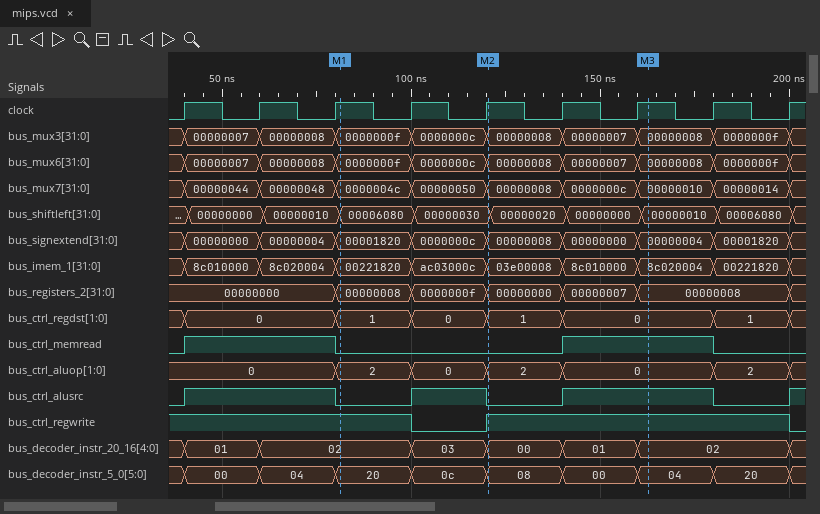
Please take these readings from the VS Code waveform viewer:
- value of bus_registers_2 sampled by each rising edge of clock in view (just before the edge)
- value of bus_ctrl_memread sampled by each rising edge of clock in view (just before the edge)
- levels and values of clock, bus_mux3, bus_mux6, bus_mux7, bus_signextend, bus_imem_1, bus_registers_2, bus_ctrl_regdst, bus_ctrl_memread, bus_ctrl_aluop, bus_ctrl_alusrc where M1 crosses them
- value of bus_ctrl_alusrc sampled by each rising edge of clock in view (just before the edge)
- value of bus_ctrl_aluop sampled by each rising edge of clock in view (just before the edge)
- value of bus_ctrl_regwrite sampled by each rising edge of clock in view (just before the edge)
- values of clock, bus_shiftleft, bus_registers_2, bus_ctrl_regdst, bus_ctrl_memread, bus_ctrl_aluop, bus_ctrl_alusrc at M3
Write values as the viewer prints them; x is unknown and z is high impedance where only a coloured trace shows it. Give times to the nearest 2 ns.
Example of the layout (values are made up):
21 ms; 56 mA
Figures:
00000000, 00000000, 00000000, 00000008, 0000000f, 00000000, 00000007, 00000008, 00000008; 0 1 1 0 0 0 1 1 0; clock=1, bus_mux3=0000000f, bus_mux6=0000000f, bus_mux7=0000004c, bus_signextend=00001820, bus_imem_1=00221820, bus_registers_2=00000008, bus_ctrl_regdst=1, bus_ctrl_memread=0, bus_ctrl_aluop=2, bus_ctrl_alusrc=0; 0 1 1 0 1 0 1 1 0; 0, 0, 0, 2, 0, 2, 0, 0, 2; 1 1 1 1 0 1 1 1 1; clock=1, bus_shiftleft=00000010, bus_registers_2=00000008, bus_ctrl_regdst=0, bus_ctrl_memread=1, bus_ctrl_aluop=0, bus_ctrl_alusrc=1
